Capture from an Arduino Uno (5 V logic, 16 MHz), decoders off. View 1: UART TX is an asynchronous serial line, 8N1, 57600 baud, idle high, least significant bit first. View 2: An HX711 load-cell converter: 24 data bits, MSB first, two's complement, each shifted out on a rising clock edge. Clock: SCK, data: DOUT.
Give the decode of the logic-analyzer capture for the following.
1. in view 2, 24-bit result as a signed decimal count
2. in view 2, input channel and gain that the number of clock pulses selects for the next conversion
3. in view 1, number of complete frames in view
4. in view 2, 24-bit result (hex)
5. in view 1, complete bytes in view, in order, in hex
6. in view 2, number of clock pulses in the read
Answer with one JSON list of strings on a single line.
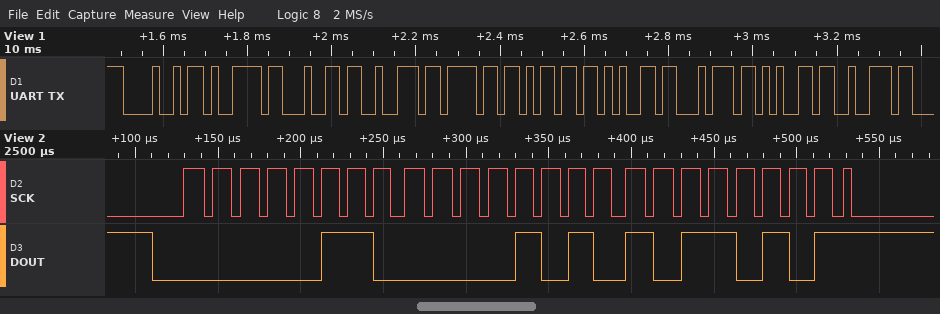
["395957", "channel A, gain 128", "10", "0x060AB5", "48 79 64 72 6F 6D 65 74 65 72", "25"]
